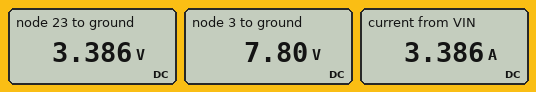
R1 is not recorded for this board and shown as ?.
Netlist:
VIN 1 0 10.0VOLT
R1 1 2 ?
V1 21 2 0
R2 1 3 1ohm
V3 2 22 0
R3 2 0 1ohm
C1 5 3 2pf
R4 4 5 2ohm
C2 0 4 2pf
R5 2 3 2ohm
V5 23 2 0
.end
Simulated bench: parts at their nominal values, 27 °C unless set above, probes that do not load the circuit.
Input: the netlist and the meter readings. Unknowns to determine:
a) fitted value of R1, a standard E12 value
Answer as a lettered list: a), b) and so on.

a) 5.6 Ω
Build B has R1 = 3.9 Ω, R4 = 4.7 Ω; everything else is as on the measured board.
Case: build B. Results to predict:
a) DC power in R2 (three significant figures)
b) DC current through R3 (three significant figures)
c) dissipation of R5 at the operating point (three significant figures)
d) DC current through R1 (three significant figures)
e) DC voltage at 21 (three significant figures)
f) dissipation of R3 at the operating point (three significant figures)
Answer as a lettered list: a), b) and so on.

a) 4.40 W
b) 3.71 A
c) 8.79 W
d) 1.61 A
e) 3.71 V
f) 13.8 W
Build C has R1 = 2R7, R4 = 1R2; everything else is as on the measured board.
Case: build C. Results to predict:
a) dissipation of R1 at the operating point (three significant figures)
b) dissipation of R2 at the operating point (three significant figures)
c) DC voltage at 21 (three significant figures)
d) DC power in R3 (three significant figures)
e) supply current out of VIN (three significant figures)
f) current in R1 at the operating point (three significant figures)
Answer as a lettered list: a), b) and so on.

a) 12.8 W
b) 3.83 W
c) 4.13 V
d) 17.1 W
e) 4.13 A
f) 2.17 A
